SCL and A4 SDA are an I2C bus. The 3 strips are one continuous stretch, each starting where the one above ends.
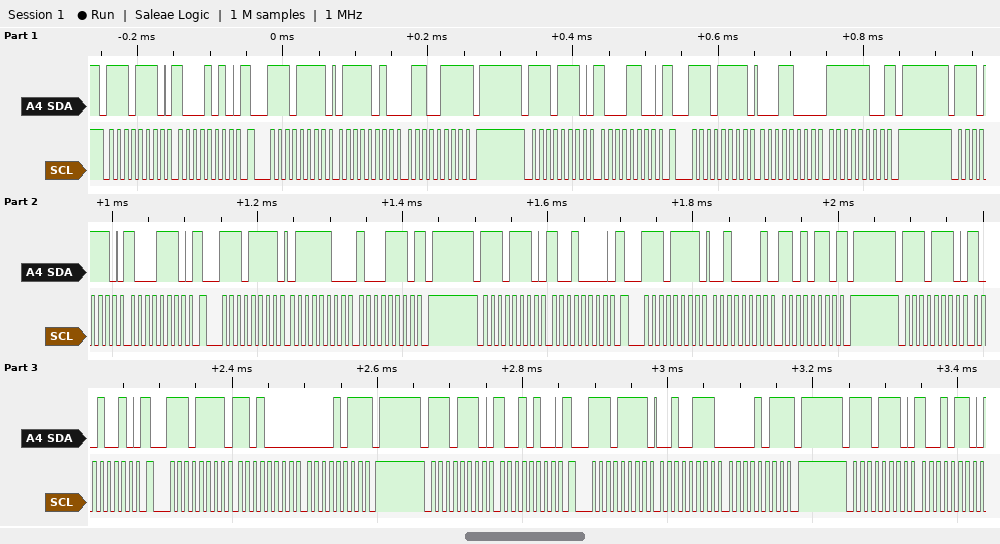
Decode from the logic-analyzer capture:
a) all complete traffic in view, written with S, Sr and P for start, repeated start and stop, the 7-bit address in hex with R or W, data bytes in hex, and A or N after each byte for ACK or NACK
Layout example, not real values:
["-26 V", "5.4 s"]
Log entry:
["S 77W A 8A A Sr 77R A 7A A 67 N P S 77W A 8C A Sr 77R A 18 A FC N P S 77W A 8E A Sr 77R A 7C A 8E N P S 77W A 90 A Sr 77R A 21 A D6 N P S 77W A 92 A Sr 77R A D0 A 0B N P S 77W A 94 A Sr 77R A 27 A 0B N P S 77W A 96 A"]
